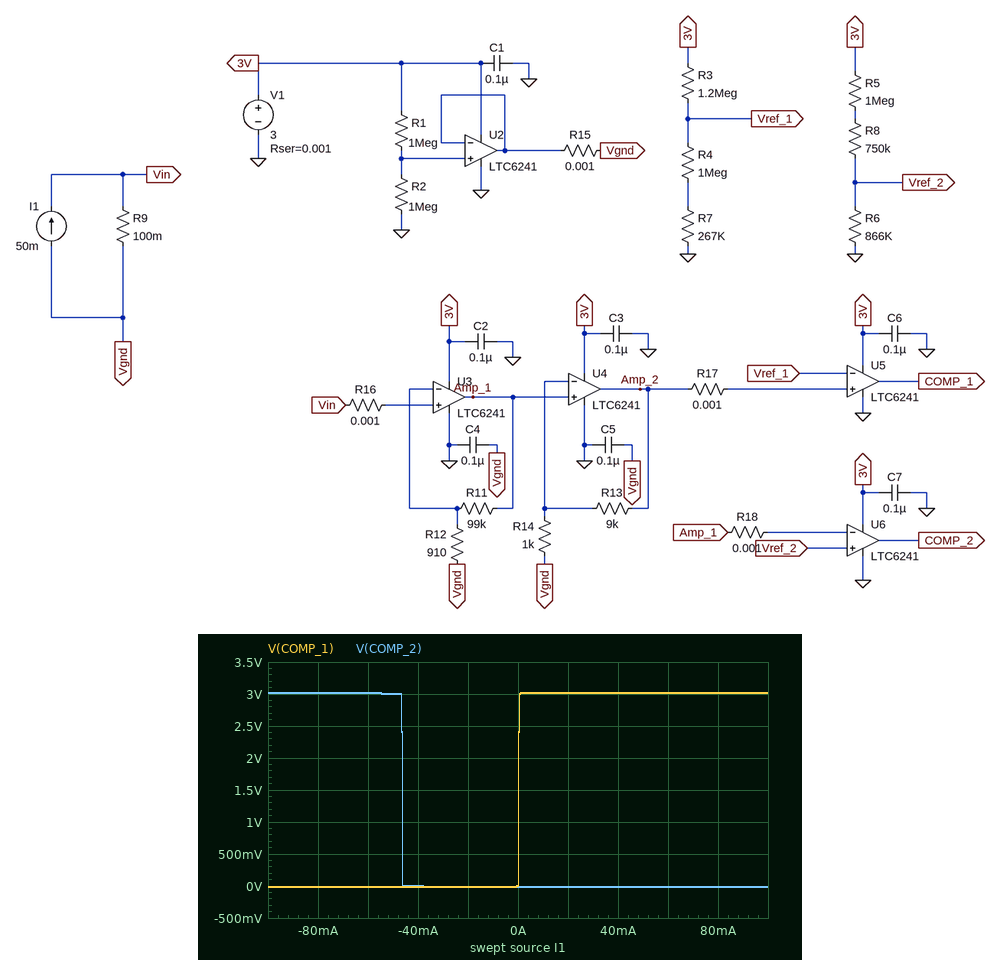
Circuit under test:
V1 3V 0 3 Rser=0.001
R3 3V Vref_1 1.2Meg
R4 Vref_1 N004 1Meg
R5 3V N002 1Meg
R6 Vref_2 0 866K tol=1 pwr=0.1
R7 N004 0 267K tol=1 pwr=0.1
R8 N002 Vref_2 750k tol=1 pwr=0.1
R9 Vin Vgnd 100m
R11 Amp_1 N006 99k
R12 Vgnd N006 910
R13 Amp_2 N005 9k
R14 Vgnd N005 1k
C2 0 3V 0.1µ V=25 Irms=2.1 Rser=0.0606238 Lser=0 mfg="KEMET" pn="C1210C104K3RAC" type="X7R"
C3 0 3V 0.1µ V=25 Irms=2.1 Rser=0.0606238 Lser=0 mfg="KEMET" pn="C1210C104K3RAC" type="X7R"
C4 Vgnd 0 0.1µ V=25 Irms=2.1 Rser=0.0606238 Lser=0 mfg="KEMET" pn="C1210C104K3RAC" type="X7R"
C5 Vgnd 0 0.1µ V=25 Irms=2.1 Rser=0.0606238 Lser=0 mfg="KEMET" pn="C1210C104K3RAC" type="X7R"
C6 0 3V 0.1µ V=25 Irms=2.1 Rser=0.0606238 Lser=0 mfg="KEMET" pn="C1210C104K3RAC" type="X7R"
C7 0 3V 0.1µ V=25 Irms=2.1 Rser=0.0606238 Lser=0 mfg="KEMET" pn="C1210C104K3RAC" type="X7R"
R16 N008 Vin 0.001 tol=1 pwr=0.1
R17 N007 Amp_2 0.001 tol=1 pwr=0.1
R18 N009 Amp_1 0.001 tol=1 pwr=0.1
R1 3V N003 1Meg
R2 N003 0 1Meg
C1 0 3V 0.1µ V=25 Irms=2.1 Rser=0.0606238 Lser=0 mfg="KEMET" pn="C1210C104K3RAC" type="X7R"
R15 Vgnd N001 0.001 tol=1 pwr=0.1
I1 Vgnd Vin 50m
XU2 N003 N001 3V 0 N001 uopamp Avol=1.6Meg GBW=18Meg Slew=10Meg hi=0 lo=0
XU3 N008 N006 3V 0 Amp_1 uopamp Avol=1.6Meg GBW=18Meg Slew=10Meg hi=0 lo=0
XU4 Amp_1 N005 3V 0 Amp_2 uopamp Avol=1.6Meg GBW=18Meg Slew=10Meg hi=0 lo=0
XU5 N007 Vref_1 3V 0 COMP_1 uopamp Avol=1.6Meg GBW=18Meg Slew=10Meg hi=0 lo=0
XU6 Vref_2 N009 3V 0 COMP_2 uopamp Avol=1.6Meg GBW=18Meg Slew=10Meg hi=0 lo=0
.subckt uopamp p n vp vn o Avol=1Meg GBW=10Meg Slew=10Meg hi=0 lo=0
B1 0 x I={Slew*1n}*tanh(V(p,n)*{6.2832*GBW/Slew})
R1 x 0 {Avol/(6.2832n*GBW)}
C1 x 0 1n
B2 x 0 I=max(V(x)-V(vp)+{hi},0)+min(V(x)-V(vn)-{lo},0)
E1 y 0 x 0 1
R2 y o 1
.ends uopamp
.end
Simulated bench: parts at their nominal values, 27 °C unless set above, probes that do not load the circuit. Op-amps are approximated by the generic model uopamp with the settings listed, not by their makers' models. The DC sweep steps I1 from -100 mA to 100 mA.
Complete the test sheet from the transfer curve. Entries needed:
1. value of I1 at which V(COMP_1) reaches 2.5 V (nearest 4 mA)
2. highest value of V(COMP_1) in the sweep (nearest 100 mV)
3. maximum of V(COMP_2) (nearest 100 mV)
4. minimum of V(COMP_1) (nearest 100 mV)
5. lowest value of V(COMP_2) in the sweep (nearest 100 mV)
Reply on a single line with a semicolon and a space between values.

0 A; 3.0 V; 3.0 V; 0 V; 0 V
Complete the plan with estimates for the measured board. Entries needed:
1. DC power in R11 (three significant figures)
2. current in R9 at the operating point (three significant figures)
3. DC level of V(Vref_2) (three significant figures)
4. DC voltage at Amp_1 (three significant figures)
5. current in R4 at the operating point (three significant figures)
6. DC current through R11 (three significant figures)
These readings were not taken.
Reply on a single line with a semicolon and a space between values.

2.99 µW; 50.0 mA; 993 mV; 2.05 V; 1.22 µA; 5.49 µA
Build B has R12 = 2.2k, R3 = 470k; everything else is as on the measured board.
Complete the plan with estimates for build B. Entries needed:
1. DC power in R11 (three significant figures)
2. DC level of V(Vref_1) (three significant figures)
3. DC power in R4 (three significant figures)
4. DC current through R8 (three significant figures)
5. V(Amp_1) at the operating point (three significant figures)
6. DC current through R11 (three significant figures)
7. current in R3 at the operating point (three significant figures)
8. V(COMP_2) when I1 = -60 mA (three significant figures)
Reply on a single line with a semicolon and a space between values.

511 nW; 2.19 V; 2.98 µW; 1.15 µA; 1.73 V; 2.27 µA; 1.73 µA; -9.89 mV
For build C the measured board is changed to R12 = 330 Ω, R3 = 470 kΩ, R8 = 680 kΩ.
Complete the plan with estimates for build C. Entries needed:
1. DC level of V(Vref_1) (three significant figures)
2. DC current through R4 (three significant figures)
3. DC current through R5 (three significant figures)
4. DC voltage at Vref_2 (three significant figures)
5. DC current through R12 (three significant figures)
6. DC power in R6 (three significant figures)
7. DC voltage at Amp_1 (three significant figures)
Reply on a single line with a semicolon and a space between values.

2.19 V; 1.73 µA; 1.18 µA; 1.02 V; 15.1 µA; 1.20 µW; 3.00 V
